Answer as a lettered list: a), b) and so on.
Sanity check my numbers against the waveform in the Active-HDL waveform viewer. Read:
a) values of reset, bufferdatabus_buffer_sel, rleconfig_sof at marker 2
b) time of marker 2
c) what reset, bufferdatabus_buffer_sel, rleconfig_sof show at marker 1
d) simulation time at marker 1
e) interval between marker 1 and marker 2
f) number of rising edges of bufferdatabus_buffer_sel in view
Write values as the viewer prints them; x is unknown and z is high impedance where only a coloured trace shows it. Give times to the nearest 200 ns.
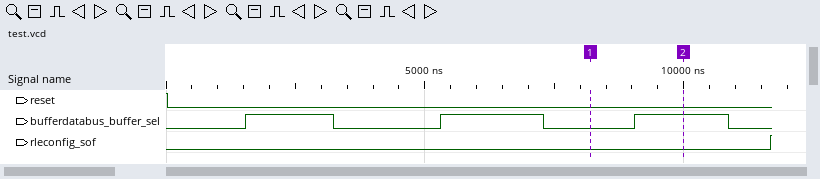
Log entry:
a) reset=0, bufferdatabus_buffer_sel=1, rleconfig_sof=0
b) 10000 ns
c) reset=0, bufferdatabus_buffer_sel=0, rleconfig_sof=0
d) 8200 ns
e) 1800 ns
f) 3
